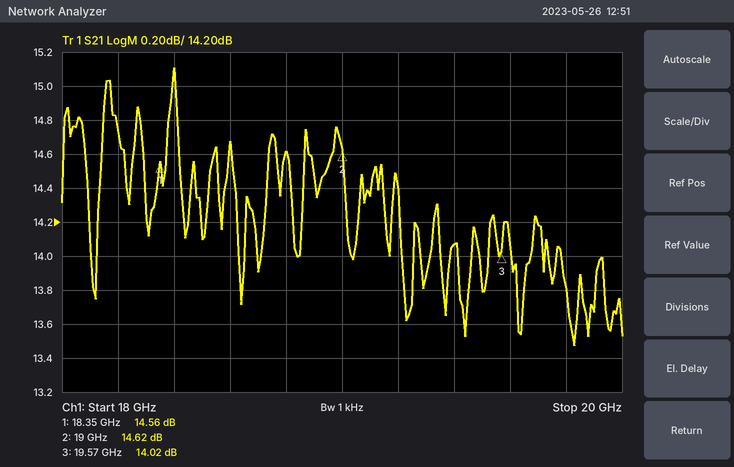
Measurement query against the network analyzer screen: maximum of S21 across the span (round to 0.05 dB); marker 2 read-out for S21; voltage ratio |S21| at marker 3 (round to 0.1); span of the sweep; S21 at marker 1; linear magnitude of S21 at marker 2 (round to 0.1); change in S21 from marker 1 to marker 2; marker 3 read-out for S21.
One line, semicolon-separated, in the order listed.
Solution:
15.10 dB; 14.62 dB; 5.0; 2 GHz; 14.56 dB; 5.4; 0.06 dB; 14.02 dB
